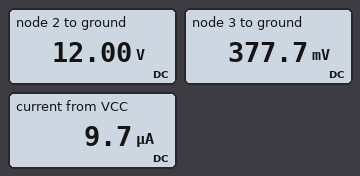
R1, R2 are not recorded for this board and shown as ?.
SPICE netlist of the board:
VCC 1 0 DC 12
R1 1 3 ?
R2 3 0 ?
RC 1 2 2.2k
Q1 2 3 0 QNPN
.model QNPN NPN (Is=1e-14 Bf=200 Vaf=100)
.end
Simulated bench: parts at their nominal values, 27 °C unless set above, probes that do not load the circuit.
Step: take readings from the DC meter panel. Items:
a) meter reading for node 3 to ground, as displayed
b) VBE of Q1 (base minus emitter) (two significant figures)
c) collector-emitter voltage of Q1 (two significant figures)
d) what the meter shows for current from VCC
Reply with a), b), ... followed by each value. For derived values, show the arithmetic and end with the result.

a) 377.7 mV
b) 377.7 mV = 380 mV
c) 12 V = 12 V
d) 9.7 µA
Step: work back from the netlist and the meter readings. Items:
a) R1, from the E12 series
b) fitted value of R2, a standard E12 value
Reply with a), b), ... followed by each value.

a) 1.2 MΩ
b) 39 kΩ
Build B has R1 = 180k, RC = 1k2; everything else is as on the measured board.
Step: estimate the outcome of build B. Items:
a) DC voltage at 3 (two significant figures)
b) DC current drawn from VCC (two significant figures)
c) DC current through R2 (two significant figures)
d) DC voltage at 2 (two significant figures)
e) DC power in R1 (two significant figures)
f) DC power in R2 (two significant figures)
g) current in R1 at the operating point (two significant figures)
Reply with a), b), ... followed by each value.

a) 710 mV
b) 9.0 mA
c) 18 µA
d) 1.3 V
e) 710 µW
f) 13 µW
g) 63 µA
